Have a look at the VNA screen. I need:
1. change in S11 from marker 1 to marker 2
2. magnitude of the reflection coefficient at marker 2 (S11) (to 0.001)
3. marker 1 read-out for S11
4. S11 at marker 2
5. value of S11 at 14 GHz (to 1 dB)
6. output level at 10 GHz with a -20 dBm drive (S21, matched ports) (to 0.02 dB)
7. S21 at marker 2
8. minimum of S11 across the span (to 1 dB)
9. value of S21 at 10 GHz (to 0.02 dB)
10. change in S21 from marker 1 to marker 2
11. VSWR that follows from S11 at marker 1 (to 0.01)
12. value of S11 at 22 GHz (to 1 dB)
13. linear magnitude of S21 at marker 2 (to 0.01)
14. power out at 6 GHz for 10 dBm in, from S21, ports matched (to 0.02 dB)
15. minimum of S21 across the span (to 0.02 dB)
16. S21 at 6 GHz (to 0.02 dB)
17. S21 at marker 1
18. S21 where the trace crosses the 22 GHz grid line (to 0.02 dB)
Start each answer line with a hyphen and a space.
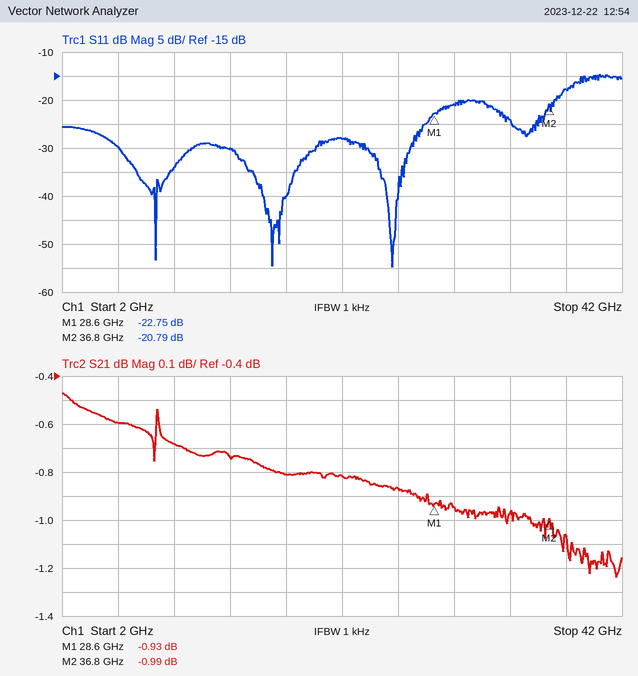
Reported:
- 1.96 dB
- 0.091
- -22.75 dB
- -20.79 dB
- -30 dB
- -20.68 dBm
- -0.99 dB
- -55 dB
- -0.68 dB
- -0.06 dB
- 1.16
- -28 dB
- 0.89
- 9.40 dBm
- -1.24 dB
- -0.60 dB
- -0.93 dB
- -0.82 dB
